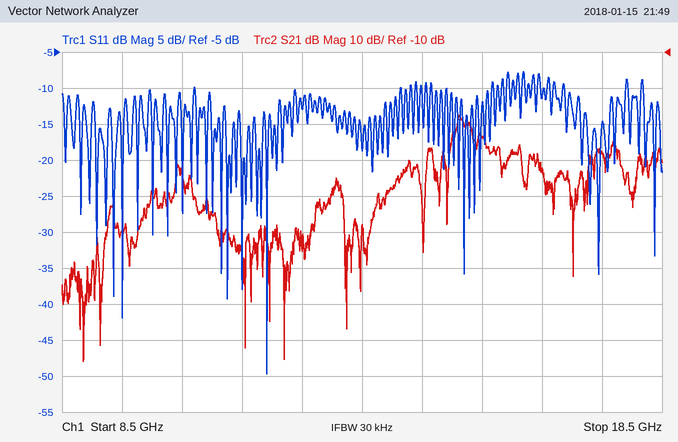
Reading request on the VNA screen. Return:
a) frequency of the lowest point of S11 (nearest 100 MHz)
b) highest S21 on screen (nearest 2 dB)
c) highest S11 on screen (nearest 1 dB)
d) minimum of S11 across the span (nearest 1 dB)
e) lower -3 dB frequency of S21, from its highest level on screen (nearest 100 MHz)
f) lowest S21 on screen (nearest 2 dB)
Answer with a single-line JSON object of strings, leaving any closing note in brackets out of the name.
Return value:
{"frequency of the lowest point of S11": "11.9 GHz", "highest S21 on screen": "-28 dB", "highest S11 on screen": "-8 dB", "minimum of S11 across the span": "-50 dB", "lower -3 dB frequency of S21, from its highest level on screen": "15.1 GHz", "lowest S21 on screen": "-96 dB"}
